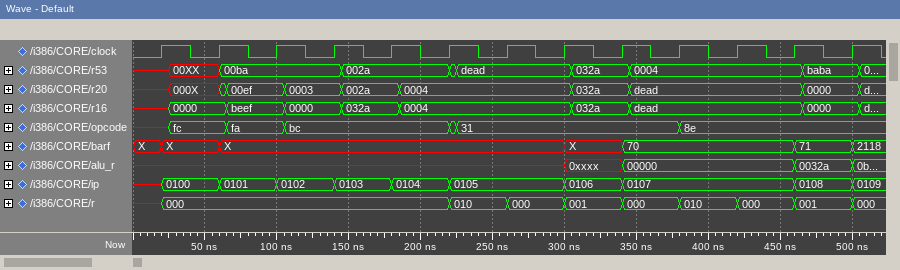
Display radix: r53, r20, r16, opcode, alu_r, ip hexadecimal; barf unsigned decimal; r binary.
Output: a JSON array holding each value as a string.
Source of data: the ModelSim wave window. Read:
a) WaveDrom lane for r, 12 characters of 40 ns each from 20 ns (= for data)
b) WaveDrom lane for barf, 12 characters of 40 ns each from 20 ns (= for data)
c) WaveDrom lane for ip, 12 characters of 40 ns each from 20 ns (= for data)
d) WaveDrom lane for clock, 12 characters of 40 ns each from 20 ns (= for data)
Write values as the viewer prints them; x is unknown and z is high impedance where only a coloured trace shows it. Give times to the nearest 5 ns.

["{name: 'r', wave: '=....=======', data: '000 010 000 001 000 010 000 001'}", "{name: 'barf', wave: '==.....==..=', data: 'X X X 70 71'}", "{name: 'ip', wave: '======.==..=', data: '0100 0101 0102 0103 0104 0105 0106 0107 0108'}", "{name: 'clock', wave: 'p...........'}"]
